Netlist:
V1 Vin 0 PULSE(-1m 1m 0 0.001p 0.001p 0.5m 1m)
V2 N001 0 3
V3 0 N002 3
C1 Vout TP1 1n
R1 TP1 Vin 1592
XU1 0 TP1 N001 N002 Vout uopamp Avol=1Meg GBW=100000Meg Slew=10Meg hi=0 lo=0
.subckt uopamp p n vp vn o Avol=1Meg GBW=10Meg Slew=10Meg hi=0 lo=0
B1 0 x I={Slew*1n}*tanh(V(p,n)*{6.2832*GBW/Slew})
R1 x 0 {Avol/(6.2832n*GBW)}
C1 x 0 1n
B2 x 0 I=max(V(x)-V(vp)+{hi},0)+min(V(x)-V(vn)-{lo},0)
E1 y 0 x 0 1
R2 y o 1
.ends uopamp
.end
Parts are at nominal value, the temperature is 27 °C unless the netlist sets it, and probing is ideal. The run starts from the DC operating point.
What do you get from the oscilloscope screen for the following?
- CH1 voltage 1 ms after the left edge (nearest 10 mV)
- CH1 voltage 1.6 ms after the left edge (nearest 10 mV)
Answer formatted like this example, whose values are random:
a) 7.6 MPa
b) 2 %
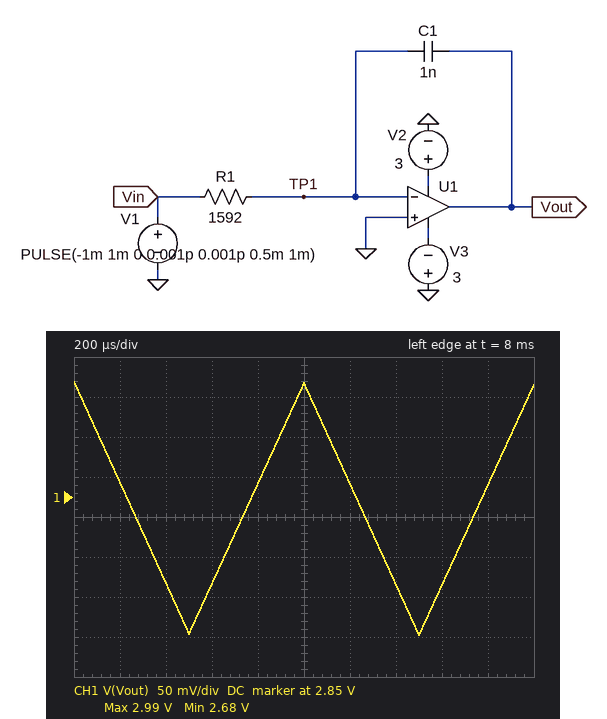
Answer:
a) 2.99 V
b) 2.74 V
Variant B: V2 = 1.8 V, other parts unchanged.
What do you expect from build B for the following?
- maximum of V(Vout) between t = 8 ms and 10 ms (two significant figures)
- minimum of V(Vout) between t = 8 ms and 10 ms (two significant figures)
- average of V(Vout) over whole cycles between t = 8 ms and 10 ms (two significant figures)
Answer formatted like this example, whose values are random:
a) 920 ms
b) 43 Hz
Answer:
a) 1.8 V
b) 1.5 V
c) 1.6 V
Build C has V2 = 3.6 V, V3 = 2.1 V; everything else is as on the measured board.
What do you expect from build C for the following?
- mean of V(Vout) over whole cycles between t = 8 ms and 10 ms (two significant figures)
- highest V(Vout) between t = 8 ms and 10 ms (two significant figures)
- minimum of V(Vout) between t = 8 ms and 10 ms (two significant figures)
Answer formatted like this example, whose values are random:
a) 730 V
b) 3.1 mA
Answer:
a) 3.4 V
b) 3.6 V
c) 3.3 V
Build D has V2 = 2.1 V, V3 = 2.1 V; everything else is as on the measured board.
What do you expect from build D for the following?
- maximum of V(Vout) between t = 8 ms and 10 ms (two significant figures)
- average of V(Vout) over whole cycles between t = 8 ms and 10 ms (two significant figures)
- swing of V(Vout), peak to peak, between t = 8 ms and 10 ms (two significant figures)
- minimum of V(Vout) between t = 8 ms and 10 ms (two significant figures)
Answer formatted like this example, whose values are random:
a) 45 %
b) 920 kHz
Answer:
a) 2.1 V
b) 1.9 V
c) 320 mV
d) 1.8 V
